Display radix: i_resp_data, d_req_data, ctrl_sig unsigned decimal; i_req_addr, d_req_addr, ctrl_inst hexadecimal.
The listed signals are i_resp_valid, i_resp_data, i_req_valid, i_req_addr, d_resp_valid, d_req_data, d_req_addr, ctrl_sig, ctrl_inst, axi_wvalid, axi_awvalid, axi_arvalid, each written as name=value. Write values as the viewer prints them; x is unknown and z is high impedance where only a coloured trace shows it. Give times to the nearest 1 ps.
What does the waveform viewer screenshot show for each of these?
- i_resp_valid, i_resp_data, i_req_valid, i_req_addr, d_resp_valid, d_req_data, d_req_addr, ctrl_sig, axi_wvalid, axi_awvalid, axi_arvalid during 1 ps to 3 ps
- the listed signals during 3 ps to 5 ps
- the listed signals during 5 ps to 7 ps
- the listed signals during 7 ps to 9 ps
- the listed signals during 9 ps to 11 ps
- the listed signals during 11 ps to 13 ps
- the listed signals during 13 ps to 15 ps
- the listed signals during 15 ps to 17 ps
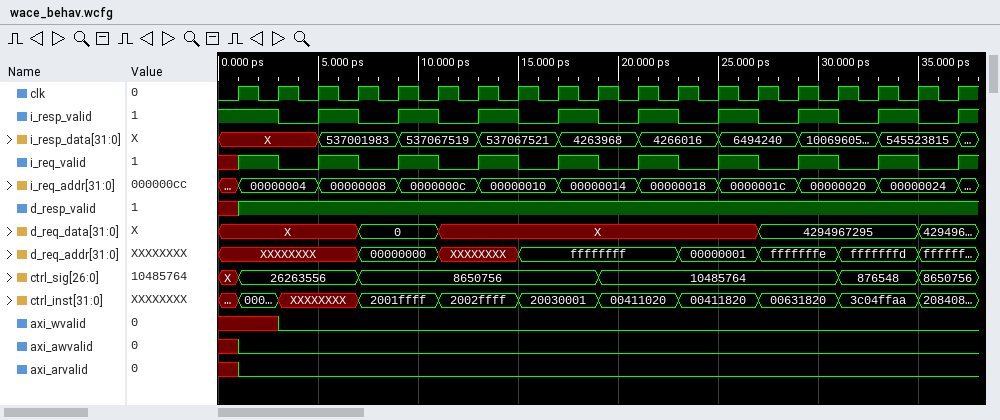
i_resp_valid=1, i_resp_data=X, i_req_valid=1, i_req_addr=00000004, d_resp_valid=1, d_req_data=X, d_req_addr=XXXXXXXX, ctrl_sig=26263556, axi_wvalid=x, axi_awvalid=0, axi_arvalid=0
i_resp_valid=0, i_resp_data=X, i_req_valid=0, i_req_addr=00000004, d_resp_valid=1, d_req_data=X, d_req_addr=XXXXXXXX, ctrl_sig=26263556, ctrl_inst=XXXXXXXX, axi_wvalid=0, axi_awvalid=0, axi_arvalid=0
i_resp_valid=1, i_resp_data=537001983, i_req_valid=1, i_req_addr=00000008, d_resp_valid=1, d_req_data=X, d_req_addr=XXXXXXXX, ctrl_sig=26263556, ctrl_inst=XXXXXXXX, axi_wvalid=0, axi_awvalid=0, axi_arvalid=0
i_resp_valid=0, i_resp_data=537001983, i_req_valid=0, i_req_addr=00000008, d_resp_valid=1, d_req_data=0, d_req_addr=00000000, ctrl_sig=8650756, ctrl_inst=2001ffff, axi_wvalid=0, axi_awvalid=0, axi_arvalid=0
i_resp_valid=1, i_resp_data=537067519, i_req_valid=1, i_req_addr=0000000c, d_resp_valid=1, d_req_data=0, d_req_addr=00000000, ctrl_sig=8650756, ctrl_inst=2001ffff, axi_wvalid=0, axi_awvalid=0, axi_arvalid=0
i_resp_valid=0, i_resp_data=537067519, i_req_valid=0, i_req_addr=0000000c, d_resp_valid=1, d_req_data=X, d_req_addr=XXXXXXXX, ctrl_sig=8650756, ctrl_inst=2002ffff, axi_wvalid=0, axi_awvalid=0, axi_arvalid=0
i_resp_valid=1, i_resp_data=537067521, i_req_valid=1, i_req_addr=00000010, d_resp_valid=1, d_req_data=X, d_req_addr=XXXXXXXX, ctrl_sig=8650756, ctrl_inst=2002ffff, axi_wvalid=0, axi_awvalid=0, axi_arvalid=0
i_resp_valid=0, i_resp_data=537067521, i_req_valid=0, i_req_addr=00000010, d_resp_valid=1, d_req_data=X, d_req_addr=ffffffff, ctrl_sig=8650756, ctrl_inst=20030001, axi_wvalid=0, axi_awvalid=0, axi_arvalid=0
